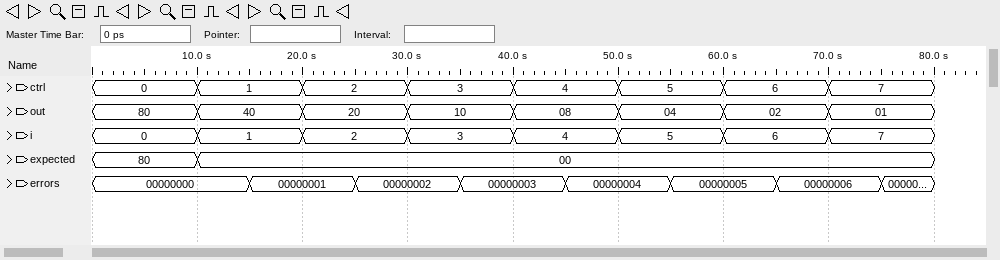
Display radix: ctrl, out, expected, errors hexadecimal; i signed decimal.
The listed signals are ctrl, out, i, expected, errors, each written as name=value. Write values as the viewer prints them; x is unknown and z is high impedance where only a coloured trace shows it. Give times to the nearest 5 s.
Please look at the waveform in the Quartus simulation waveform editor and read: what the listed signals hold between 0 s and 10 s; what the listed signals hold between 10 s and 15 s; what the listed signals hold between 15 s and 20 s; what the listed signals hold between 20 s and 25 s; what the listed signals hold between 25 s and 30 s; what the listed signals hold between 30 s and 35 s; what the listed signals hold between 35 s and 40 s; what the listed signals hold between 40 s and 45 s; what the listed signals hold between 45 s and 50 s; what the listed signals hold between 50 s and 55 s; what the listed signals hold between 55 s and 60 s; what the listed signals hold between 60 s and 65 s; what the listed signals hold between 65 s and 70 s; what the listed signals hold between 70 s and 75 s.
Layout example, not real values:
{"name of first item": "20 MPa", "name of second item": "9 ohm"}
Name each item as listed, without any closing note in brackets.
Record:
{"what the listed signals hold between 0 s and 10 s": "ctrl=0, out=80, i=0, expected=80, errors=00000000", "what the listed signals hold between 10 s and 15 s": "ctrl=1, out=40, i=1, expected=00, errors=00000000", "what the listed signals hold between 15 s and 20 s": "ctrl=1, out=40, i=1, expected=00, errors=00000001", "what the listed signals hold between 20 s and 25 s": "ctrl=2, out=20, i=2, expected=00, errors=00000001", "what the listed signals hold between 25 s and 30 s": "ctrl=2, out=20, i=2, expected=00, errors=00000002", "what the listed signals hold between 30 s and 35 s": "ctrl=3, out=10, i=3, expected=00, errors=00000002", "what the listed signals hold between 35 s and 40 s": "ctrl=3, out=10, i=3, expected=00, errors=00000003", "what the listed signals hold between 40 s and 45 s": "ctrl=4, out=08, i=4, expected=00, errors=00000003", "what the listed signals hold between 45 s and 50 s": "ctrl=4, out=08, i=4, expected=00, errors=00000004", "what the listed signals hold between 50 s and 55 s": "ctrl=5, out=04, i=5, expected=00, errors=00000004", "what the listed signals hold between 55 s and 60 s": "ctrl=5, out=04, i=5, expected=00, errors=00000005", "what the listed signals hold between 60 s and 65 s": "ctrl=6, out=02, i=6, expected=00, errors=00000005", "what the listed signals hold between 65 s and 70 s": "ctrl=6, out=02, i=6, expected=00, errors=00000006", "what the listed signals hold between 70 s and 75 s": "ctrl=7, out=01, i=7, expected=00, errors=00000006"}
